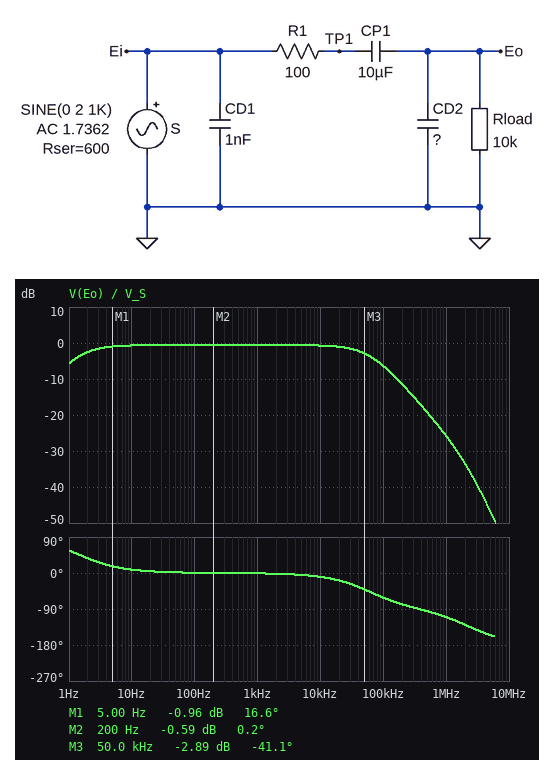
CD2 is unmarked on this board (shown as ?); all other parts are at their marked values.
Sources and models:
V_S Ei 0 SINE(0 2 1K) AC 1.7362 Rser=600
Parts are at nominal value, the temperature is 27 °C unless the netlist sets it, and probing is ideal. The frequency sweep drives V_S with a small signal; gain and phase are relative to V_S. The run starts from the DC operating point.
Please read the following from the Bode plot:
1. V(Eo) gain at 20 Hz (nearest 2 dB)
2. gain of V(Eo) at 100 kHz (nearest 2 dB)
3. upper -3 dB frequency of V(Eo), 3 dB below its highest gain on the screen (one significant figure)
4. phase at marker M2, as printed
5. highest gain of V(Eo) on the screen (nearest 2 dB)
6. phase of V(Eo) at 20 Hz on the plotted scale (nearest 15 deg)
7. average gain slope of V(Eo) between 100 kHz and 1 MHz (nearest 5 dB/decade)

0 dB
-6 dB
60 kHz
0.2 deg
0 dB
0 deg
-20 dB/decade
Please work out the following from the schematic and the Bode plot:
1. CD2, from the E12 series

3.3 nF
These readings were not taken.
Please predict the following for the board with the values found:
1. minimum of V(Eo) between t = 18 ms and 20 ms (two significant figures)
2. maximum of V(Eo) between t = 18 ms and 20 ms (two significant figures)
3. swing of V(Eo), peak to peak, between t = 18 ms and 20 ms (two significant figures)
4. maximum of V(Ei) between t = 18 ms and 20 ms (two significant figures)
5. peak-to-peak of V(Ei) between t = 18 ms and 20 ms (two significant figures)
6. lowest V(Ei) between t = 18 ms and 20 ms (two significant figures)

-1.9 V
1.9 V
3.7 V
1.9 V
3.8 V
-1.9 V
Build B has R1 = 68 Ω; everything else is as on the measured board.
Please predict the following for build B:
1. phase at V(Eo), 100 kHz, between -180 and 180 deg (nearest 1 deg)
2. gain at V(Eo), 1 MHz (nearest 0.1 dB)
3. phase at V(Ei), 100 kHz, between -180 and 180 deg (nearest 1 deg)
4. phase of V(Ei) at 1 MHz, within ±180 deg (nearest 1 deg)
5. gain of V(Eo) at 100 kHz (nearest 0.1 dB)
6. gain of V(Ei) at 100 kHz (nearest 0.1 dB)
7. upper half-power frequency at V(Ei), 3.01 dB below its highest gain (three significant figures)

-60 deg
-25.2 dB
-52 deg
-49 deg
-6.2 dB
-6.0 dB
54.8 kHz
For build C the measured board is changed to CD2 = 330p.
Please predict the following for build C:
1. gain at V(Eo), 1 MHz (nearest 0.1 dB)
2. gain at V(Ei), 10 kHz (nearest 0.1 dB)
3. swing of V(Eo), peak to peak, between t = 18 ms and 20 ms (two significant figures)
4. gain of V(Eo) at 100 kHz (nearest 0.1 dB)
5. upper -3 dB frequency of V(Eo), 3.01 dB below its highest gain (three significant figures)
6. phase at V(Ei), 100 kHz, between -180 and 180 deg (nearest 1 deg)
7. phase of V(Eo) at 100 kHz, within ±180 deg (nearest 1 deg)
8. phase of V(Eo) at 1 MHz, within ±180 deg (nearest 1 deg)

-14.4 dB
-0.5 dB
3.7 V
-1.5 dB
210 kHz
-25 deg
-26 deg
-87 deg
